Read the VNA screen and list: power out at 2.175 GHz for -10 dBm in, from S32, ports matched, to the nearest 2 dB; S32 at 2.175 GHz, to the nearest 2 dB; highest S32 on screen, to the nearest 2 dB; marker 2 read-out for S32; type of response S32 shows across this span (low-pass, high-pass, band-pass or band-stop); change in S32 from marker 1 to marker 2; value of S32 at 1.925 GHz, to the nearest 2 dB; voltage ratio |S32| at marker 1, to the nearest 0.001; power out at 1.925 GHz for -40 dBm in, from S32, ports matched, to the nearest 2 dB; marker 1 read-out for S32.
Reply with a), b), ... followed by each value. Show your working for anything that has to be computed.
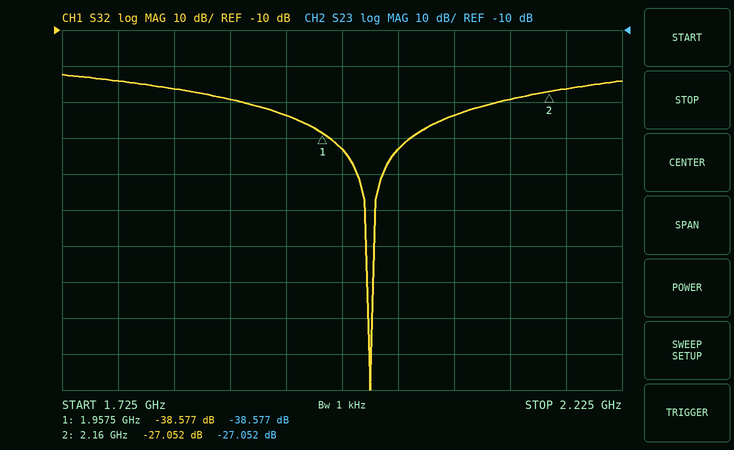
a) -10 dBm + (-26 dB) = -36 dBm
b) -26 dB
c) -22 dB
d) -27.052 dB
e) band-stop
f) -27.052 − (-38.577) = 11.525 dB
g) -34 dB
h) 10^(-38.577/20) ≈ 0.012
i) -40 dBm + (-34 dB) = -74 dBm
j) -38.577 dB
